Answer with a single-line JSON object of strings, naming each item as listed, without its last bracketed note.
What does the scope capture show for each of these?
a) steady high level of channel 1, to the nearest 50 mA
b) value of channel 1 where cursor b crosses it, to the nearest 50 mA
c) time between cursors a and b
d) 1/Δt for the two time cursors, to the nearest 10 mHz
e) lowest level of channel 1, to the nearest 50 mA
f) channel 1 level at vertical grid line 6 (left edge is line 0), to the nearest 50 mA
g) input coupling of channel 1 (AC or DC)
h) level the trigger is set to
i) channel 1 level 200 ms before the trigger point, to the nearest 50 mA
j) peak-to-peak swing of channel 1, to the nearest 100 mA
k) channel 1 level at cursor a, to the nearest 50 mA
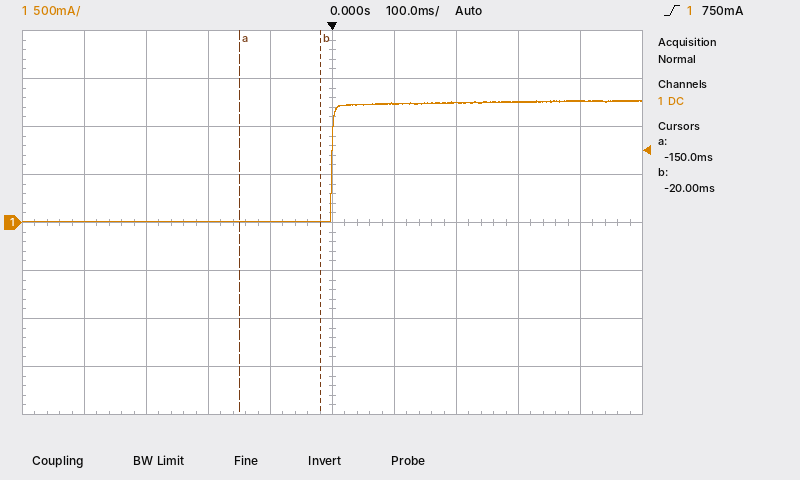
{"steady high level of channel 1, to the nearest 50 mA": "1.25 A", "value of channel 1 where cursor b crosses it, to the nearest 50 mA": "0 mA", "time between cursors a and b": "130 ms", "1/Δt for the two time cursors, to the nearest 10 mHz": "7.69 Hz", "lowest level of channel 1, to the nearest 50 mA": "0 mA", "channel 1 level at vertical grid line 6 (left edge is line 0), to the nearest 50 mA": "1.25 A", "input coupling of channel 1": "DC", "level the trigger is set to": "750 mA", "channel 1 level 200 ms before the trigger point, to the nearest 50 mA": "0 mA", "peak-to-peak swing of channel 1, to the nearest 100 mA": "1.30 A", "channel 1 level at cursor a, to the nearest 50 mA": "0 mA"}
